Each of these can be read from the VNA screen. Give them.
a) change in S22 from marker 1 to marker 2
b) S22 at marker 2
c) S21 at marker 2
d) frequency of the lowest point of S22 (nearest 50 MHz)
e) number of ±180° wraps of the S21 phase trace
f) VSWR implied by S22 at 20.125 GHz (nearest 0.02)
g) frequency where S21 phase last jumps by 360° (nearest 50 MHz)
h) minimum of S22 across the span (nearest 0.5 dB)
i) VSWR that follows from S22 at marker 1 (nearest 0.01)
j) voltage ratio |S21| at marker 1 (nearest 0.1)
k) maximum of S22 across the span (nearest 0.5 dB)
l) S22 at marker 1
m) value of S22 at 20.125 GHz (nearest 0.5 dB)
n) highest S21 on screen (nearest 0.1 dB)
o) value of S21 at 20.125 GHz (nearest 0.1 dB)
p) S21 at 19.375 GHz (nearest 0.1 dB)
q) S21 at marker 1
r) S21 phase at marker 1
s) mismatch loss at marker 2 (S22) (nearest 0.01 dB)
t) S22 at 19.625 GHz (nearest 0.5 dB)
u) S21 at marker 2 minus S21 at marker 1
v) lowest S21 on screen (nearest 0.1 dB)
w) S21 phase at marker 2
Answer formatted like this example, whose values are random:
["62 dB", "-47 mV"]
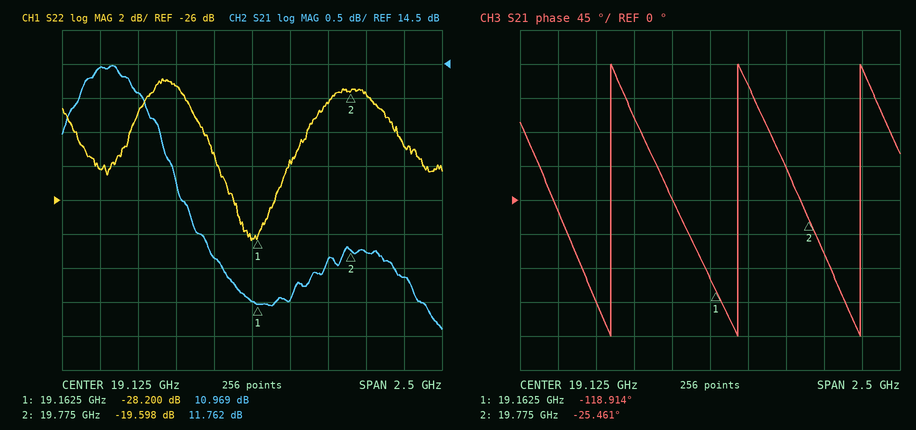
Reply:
["8.602 dB", "-19.598 dB", "11.762 dB", "19.10 GHz", "3", "1.16", "20.10 GHz", "-28.5 dB", "1.08", "3.5", "-19.0 dB", "-28.200 dB", "-23.0 dB", "14.5 dB", "11.4 dB", "11.0 dB", "10.969 dB", "-118.914°", "0.05 dB", "-20.5 dB", "0.793 dB", "10.6 dB", "-25.461°"]
